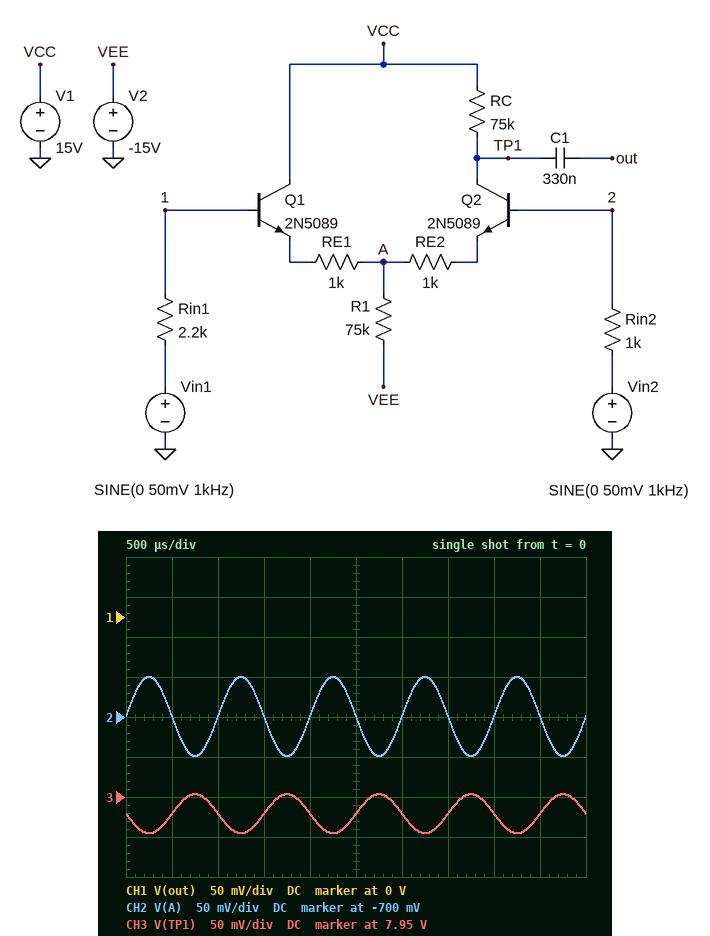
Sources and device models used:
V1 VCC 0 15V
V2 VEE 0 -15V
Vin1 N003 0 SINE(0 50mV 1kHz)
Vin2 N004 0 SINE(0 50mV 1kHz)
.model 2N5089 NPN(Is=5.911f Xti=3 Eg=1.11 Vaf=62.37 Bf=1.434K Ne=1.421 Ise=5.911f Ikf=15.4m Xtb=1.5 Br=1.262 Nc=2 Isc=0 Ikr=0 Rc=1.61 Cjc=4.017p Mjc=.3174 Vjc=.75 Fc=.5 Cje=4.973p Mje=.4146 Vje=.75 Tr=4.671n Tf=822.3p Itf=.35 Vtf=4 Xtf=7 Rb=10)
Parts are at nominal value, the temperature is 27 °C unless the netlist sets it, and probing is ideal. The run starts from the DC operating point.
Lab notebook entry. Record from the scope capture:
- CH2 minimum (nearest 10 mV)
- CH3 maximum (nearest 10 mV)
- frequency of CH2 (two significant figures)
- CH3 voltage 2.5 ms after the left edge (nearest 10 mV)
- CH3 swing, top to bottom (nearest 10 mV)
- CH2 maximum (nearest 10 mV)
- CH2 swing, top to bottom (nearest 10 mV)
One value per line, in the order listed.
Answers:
-750 mV
7.95 V
1.0 kHz
7.93 V
50 mV
-650 mV
100 mV
